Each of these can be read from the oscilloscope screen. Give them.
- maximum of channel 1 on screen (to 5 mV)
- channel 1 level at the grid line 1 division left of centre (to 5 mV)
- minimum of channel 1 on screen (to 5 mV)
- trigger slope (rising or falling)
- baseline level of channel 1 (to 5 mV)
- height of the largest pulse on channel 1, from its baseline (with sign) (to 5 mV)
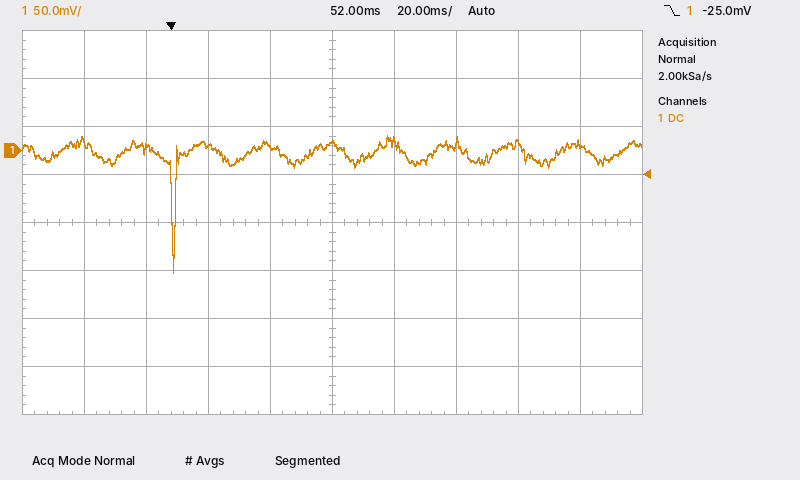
15 mV
5 mV
-125 mV
falling
0 mV
-125 mV
